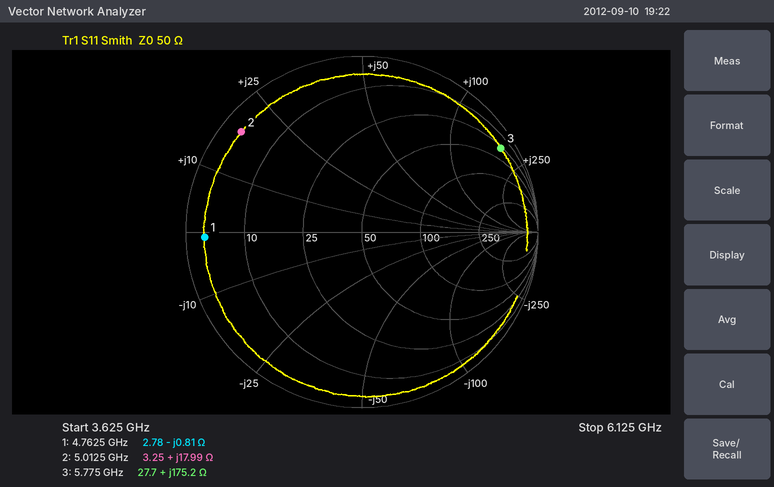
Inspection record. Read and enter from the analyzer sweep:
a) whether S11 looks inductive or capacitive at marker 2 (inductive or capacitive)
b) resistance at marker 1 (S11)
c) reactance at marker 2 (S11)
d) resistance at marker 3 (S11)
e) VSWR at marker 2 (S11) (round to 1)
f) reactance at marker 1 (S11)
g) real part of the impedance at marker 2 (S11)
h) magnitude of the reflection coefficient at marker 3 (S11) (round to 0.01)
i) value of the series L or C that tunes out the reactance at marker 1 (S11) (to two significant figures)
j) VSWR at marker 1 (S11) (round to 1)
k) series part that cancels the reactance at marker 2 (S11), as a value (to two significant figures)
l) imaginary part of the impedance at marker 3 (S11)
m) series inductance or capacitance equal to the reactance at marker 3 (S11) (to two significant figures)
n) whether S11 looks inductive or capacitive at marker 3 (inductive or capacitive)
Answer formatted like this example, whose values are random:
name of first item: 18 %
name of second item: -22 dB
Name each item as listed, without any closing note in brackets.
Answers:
whether S11 looks inductive or capacitive at marker 2: inductive
resistance at marker 1: 2.78 Ω
reactance at marker 2: +17.99 Ω
resistance at marker 3: 27.7 Ω
VSWR at marker 2 (S11): 17
reactance at marker 1: -0.81 Ω
real part of the impedance at marker 2: 3.25 Ω
magnitude of the reflection coefficient at marker 3 (S11): 0.92
value of the series L or C that tunes out the reactance at marker 1 (S11): 27 pH
VSWR at marker 1 (S11): 18
series part that cancels the reactance at marker 2 (S11), as a value: 1.8 pF
imaginary part of the impedance at marker 3: +175.2 Ω
series inductance or capacitance equal to the reactance at marker 3 (S11): 4.8 nH
whether S11 looks inductive or capacitive at marker 3: inductive
